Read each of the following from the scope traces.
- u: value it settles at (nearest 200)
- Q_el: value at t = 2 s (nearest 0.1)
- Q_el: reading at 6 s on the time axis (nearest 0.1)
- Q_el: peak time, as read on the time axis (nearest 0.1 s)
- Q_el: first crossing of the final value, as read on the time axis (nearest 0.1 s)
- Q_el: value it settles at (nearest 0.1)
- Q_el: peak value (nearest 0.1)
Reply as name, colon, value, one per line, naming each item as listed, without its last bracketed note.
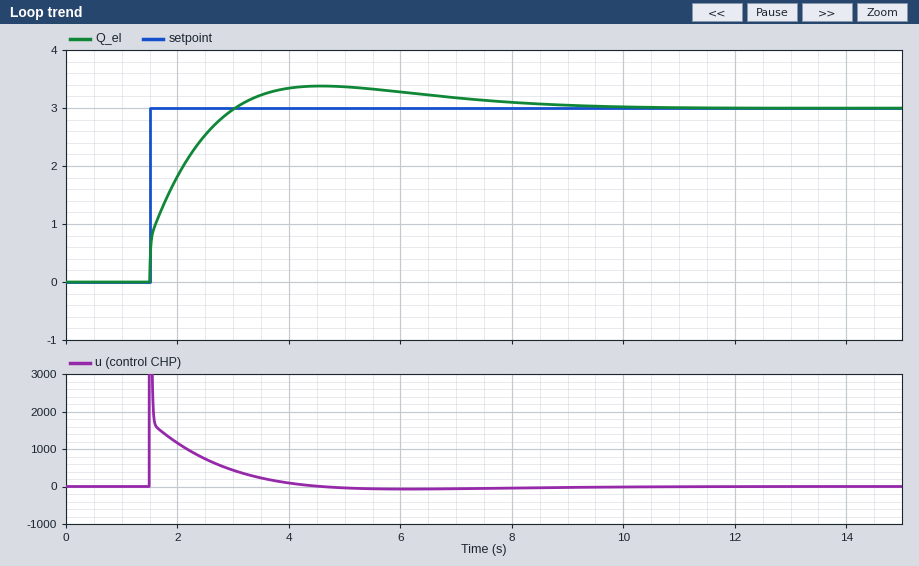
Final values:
u: value it settles at: 0
Q_el: value at t = 2 s: 1.8
Q_el: reading at 6 s on the time axis: 3.3
Q_el: peak time, as read on the time axis: 4.6 s
Q_el: first crossing of the final value, as read on the time axis: 3.0 s
Q_el: value it settles at: 3.0
Q_el: peak value: 3.4
